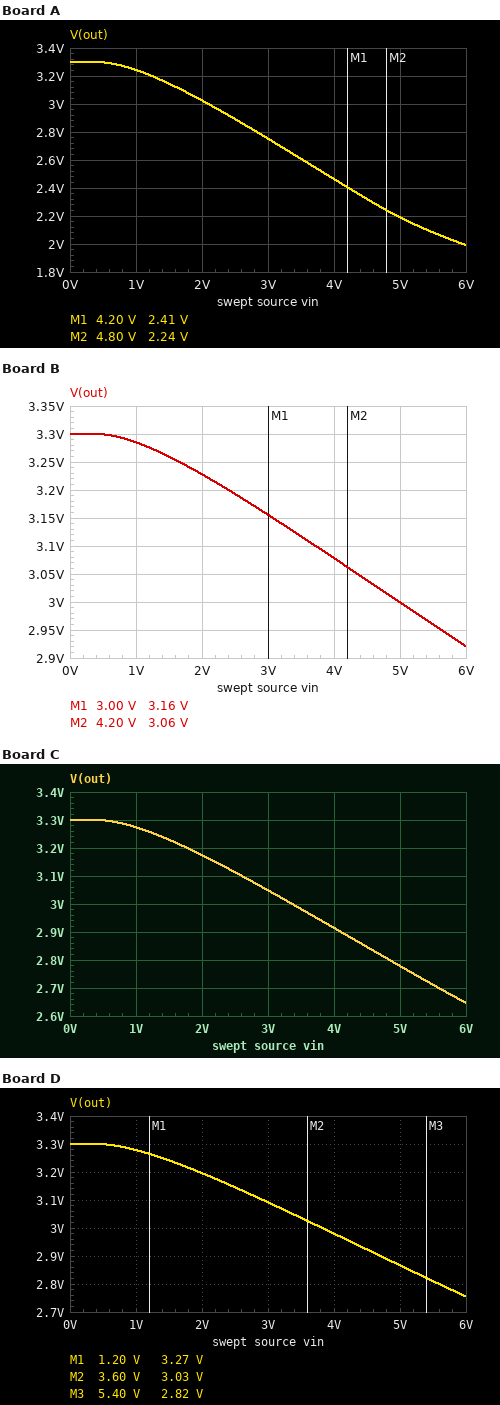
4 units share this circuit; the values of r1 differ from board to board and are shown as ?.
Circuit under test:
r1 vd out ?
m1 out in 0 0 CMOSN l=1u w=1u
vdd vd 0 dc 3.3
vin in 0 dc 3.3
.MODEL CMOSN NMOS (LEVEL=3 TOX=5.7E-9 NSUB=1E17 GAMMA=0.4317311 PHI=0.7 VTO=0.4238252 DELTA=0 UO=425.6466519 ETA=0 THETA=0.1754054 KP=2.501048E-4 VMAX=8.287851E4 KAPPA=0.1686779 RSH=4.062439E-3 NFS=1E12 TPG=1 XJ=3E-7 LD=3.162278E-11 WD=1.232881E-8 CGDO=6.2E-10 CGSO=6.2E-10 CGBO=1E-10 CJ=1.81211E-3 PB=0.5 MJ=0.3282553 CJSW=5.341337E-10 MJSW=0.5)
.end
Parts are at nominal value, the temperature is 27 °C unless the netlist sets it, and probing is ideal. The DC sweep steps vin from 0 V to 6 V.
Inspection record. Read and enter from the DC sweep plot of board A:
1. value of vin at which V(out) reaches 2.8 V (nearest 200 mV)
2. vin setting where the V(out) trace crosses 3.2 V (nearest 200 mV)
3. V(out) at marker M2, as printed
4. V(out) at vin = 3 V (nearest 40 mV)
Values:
2.8 V
1.2 V
2.24 V
2.76 V
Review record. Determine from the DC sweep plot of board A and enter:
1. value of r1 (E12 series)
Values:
1.8 kΩ
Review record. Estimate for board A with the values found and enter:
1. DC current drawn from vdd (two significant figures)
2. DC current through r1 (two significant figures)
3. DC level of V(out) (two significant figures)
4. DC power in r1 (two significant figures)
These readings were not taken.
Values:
350 µA
350 µA
2.7 V
220 µW
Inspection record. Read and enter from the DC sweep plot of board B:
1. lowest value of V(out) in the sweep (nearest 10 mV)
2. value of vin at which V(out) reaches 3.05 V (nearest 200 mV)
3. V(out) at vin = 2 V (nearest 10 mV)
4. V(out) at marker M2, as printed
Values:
2.92 V
4.4 V
3.23 V
3.06 V
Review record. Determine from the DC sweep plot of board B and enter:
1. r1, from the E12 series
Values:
470 Ω
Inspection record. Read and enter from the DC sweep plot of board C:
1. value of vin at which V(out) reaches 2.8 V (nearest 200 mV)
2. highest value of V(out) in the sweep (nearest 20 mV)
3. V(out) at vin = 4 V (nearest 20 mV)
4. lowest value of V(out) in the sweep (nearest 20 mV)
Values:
4.8 V
3.30 V
2.92 V
2.64 V
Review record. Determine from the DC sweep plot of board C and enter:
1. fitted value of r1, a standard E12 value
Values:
820 Ω
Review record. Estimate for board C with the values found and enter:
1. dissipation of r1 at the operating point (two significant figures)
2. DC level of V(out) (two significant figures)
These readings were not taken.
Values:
100 µW
3.0 V
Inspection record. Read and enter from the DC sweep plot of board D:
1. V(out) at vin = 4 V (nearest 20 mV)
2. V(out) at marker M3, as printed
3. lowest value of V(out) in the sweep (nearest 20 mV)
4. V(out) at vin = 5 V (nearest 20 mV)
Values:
2.98 V
2.82 V
2.76 V
2.86 V
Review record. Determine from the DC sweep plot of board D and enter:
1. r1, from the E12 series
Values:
680 Ω
